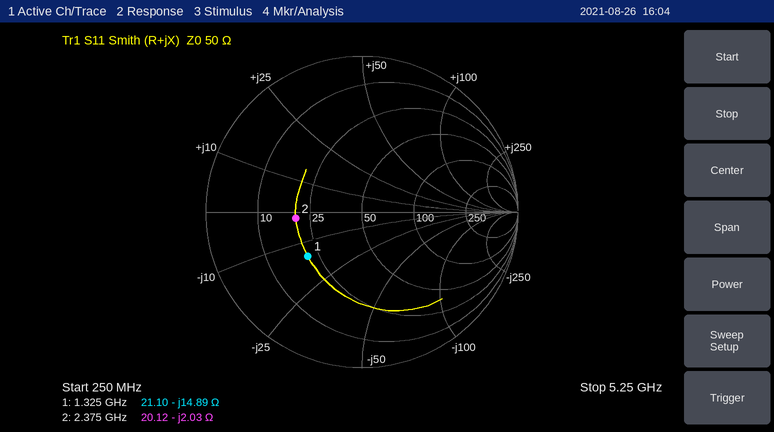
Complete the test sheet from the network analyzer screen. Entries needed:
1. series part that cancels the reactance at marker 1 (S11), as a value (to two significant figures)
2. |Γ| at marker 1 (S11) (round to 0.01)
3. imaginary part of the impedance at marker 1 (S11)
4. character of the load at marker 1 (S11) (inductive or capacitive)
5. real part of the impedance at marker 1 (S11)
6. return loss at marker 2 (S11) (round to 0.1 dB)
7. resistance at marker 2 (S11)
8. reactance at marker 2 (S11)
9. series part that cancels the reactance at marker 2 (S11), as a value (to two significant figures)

1.8 nH
0.45
-14.89 Ω
capacitive
21.10 Ω
7.4 dB
20.12 Ω
-2.03 Ω
140 pH
